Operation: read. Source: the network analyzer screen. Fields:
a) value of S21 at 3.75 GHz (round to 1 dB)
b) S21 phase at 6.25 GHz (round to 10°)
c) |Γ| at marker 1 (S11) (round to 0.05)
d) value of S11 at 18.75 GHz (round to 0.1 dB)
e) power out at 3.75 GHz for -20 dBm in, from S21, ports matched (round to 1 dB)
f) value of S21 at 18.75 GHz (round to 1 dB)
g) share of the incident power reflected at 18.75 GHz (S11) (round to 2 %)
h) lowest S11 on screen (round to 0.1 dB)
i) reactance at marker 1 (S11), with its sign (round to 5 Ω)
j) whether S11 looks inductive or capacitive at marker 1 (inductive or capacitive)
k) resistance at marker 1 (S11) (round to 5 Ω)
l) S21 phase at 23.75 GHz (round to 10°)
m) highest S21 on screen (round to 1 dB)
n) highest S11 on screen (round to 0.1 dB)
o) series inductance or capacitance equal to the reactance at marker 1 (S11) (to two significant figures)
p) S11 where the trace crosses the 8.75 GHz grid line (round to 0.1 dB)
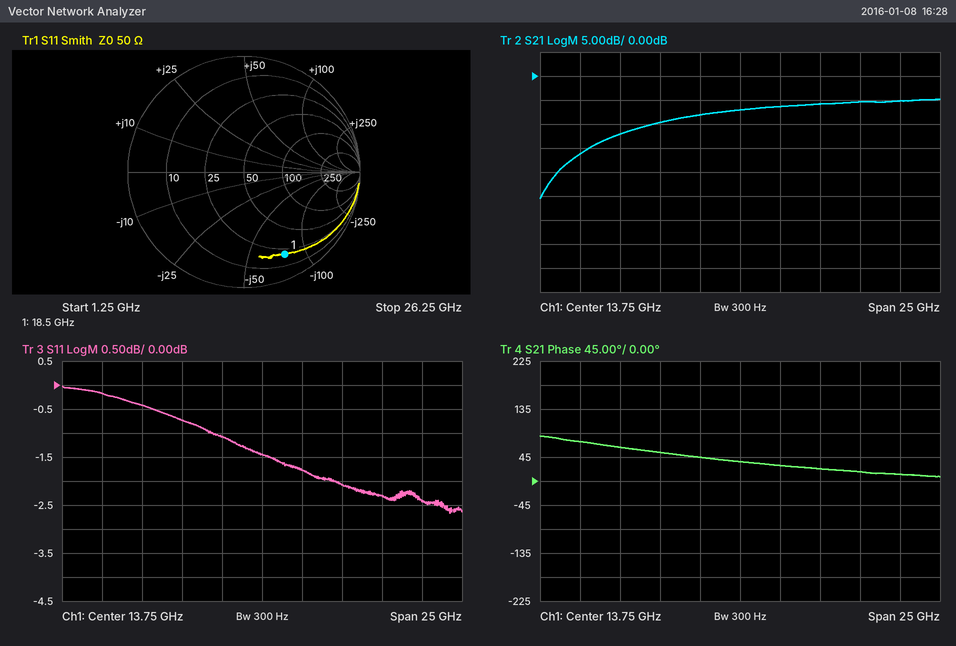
-16 dB
60°
0.80
-2.1 dB
-36 dBm
-6 dB
62 %
-2.7 dB
-75 Ω
capacitive
20 Ω
10°
-5 dB
0.0 dB
110 fF
-0.7 dB
